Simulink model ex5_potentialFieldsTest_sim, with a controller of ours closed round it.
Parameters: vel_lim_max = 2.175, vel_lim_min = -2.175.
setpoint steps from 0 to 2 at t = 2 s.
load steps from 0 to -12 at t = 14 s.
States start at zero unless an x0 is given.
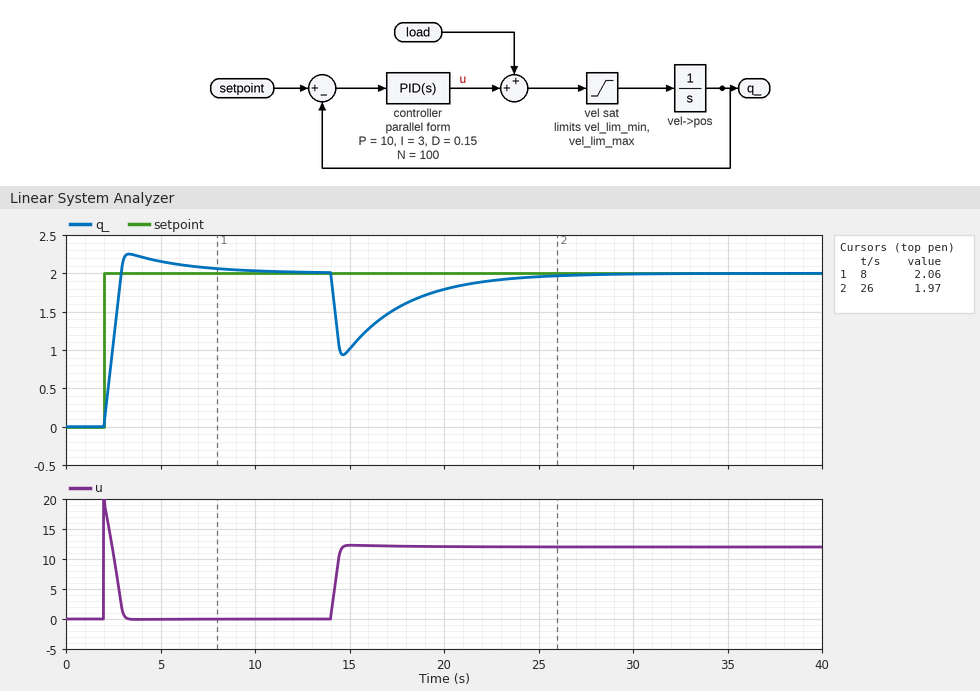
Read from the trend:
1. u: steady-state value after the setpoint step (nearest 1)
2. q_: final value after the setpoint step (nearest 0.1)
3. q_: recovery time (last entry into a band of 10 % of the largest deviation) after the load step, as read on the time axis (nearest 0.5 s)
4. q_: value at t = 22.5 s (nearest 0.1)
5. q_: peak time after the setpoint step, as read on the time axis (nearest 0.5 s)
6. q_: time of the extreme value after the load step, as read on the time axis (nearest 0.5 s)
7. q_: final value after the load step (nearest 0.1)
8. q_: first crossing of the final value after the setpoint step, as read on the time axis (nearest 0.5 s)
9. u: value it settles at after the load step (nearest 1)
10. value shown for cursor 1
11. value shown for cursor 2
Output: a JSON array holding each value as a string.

["0", "2.0", "22.0 s", "1.9", "3.5 s", "14.5 s", "2.0", "3.0 s", "12", "2.06", "1.97"]
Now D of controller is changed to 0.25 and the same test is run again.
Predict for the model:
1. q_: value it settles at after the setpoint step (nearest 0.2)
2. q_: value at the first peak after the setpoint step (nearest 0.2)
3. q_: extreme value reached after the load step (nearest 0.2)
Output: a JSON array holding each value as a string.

["2.0", "2.2", "1.0"]
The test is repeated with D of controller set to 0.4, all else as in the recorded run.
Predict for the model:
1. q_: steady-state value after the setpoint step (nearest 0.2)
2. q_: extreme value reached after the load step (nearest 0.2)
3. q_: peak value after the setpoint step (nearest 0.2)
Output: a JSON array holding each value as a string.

["2.0", "1.0", "2.2"]
